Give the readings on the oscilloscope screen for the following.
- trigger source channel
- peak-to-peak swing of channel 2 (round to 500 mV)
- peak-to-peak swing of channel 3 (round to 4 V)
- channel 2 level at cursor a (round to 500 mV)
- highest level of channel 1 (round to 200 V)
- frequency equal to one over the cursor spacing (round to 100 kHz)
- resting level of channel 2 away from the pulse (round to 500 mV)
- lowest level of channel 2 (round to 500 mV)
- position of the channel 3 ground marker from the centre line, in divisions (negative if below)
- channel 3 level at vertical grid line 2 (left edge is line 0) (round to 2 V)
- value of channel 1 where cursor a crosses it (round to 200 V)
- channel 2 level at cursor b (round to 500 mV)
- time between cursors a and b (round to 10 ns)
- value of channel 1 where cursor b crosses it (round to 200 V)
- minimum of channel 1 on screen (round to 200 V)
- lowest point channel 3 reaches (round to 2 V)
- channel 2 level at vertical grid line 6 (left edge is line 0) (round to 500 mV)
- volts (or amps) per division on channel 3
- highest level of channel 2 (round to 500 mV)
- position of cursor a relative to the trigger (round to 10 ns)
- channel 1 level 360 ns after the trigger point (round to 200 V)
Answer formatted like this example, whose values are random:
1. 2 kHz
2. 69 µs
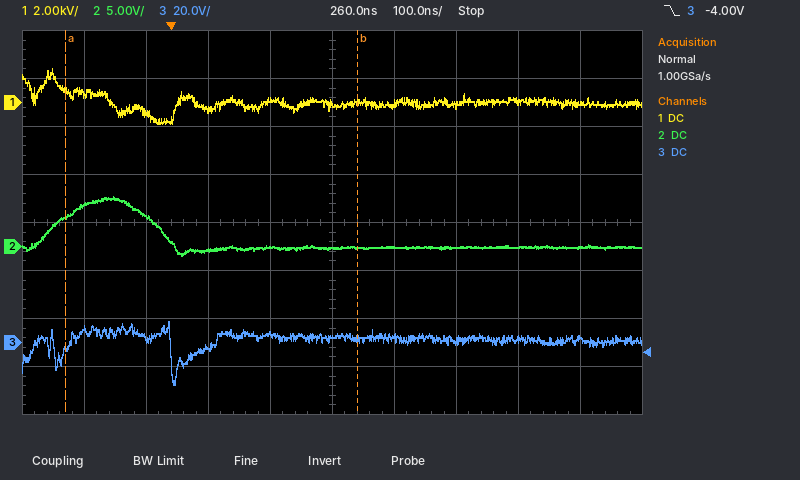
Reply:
1. channel 3
2. 6.0 V
3. 28 V
4. 3.0 V
5. 1.4 kV
6. 2.1 MHz
7. 0.0 V
8. -1.0 V
9. -2.5 div
10. 2 V
11. 600 V
12. 0.0 V
13. 470 ns
14. 0.0 kV
15. -800 V
16. -18 V
17. 0.0 V
18. 20 V
19. 5.0 V
20. -170 ns
21. 0.0 kV
